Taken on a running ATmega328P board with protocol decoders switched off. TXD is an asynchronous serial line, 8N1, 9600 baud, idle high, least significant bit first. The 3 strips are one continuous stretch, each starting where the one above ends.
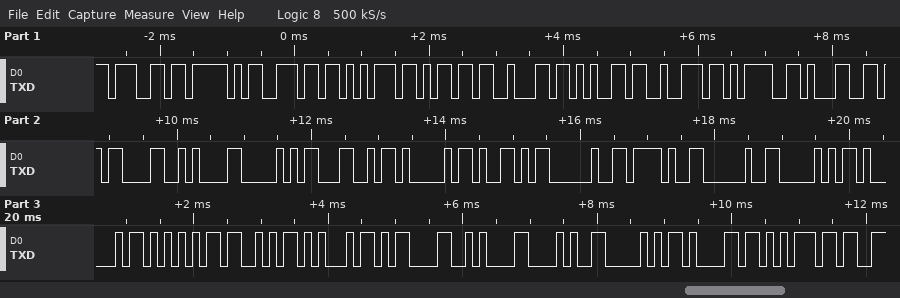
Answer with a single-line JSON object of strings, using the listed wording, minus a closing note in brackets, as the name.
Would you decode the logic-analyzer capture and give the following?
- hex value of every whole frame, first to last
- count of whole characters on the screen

{"hex value of every whole frame, first to last": "67 5F 6E 75 6D 62 65 72 3D 31 0D 0A 50 4C 41 59 20 2F 20 50 41 55 53 45 0D 0A 28 50 61 75", "count of whole characters on the screen": "30"}
